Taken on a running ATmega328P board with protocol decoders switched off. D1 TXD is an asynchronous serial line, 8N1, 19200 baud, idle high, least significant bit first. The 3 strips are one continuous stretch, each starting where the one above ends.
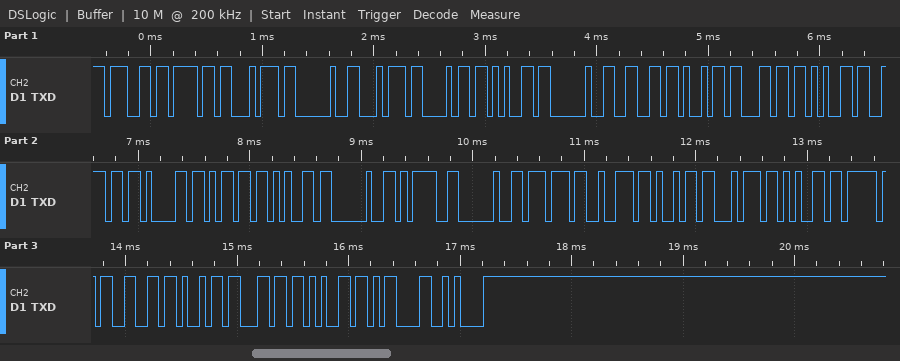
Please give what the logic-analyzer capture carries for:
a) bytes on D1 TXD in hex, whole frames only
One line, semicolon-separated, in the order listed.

67 6F 74 20 74 68 65 20 66 69 6C 65 6E 61 6D 65 20 3D 20 77 72 69 74 65 5F 66 69 6C 65 0D 0A
